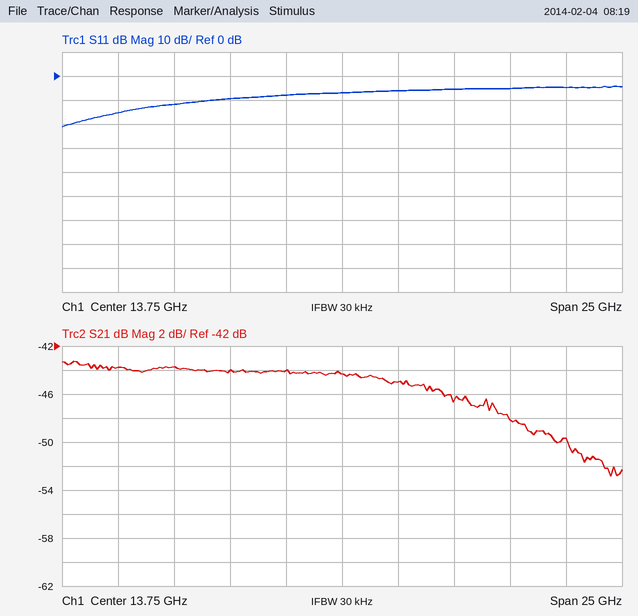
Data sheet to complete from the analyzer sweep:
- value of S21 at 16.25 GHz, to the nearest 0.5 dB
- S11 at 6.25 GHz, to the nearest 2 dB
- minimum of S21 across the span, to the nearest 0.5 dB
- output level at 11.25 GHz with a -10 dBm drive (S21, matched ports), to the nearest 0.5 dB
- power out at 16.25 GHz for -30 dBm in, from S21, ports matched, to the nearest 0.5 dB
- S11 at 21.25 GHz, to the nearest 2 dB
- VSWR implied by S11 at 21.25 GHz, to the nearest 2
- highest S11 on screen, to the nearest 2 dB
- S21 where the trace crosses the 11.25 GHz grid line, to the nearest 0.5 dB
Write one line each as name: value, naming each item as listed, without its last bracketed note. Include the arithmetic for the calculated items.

value of S21 at 16.25 GHz, to the nearest 0.5 dB: -45.0 dB
S11 at 6.25 GHz, to the nearest 2 dB: -12 dB
minimum of S21 across the span, to the nearest 0.5 dB: -53.0 dB
output level at 11.25 GHz with a -10 dBm drive (S21, matched ports), to the nearest 0.5 dB: -10 dBm + (-44.0 dB) = -54.0 dBm
power out at 16.25 GHz for -30 dBm in, from S21, ports matched, to the nearest 0.5 dB: -30 dBm + (-45.0 dB) = -75.0 dBm
S11 at 21.25 GHz, to the nearest 2 dB: -6 dB
VSWR implied by S11 at 21.25 GHz, to the nearest 2: |Γ| = 10^(-6/20) = 0.5012; VSWR = (1 + 0.5012)/(1 − 0.5012) ≈ 3.01, so 4 to the nearest 2
highest S11 on screen, to the nearest 2 dB: -4 dB
S21 where the trace crosses the 11.25 GHz grid line, to the nearest 0.5 dB: -44.0 dB
